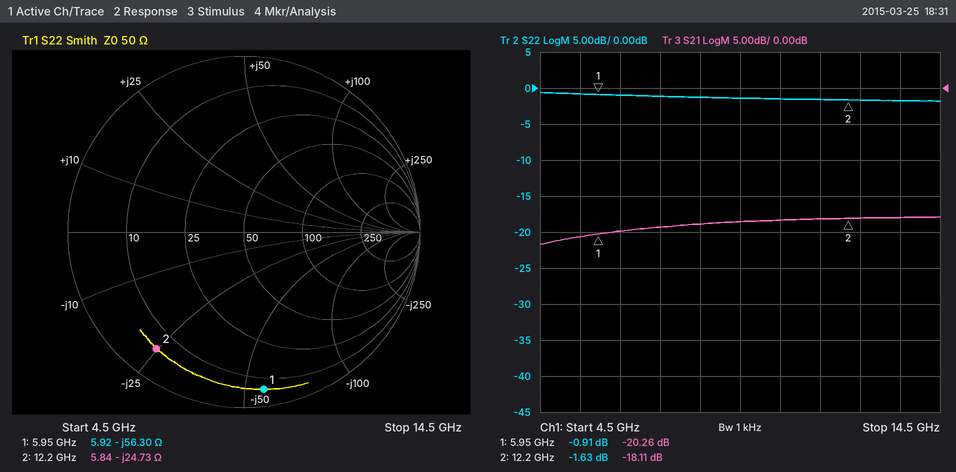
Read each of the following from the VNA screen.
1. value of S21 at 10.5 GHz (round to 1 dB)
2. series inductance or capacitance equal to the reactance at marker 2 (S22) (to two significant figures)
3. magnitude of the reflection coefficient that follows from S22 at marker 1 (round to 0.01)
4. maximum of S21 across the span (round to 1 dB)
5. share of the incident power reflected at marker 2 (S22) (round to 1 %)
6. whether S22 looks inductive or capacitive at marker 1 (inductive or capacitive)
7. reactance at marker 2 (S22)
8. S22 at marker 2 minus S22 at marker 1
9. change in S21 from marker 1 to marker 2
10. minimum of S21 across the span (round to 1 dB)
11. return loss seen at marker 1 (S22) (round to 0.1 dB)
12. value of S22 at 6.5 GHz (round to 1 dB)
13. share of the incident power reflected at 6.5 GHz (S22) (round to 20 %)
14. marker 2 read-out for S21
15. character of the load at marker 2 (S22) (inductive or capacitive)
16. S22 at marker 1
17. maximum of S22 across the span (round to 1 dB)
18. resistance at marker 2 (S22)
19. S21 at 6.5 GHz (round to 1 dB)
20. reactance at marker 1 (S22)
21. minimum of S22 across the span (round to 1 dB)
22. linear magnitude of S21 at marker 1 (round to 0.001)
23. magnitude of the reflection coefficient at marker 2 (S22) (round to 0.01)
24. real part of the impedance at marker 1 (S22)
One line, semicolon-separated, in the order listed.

-18 dB; 530 fF; 0.90; -18 dB; 69 %; capacitive; -24.73 Ω; -0.72 dB; 2.15 dB; -22 dB; 0.9 dB; -1 dB; 80 %; -18.11 dB; capacitive; -0.91 dB; -1 dB; 5.84 Ω; -20 dB; -56.30 Ω; -2 dB; 0.097; 0.83; 5.92 Ω
